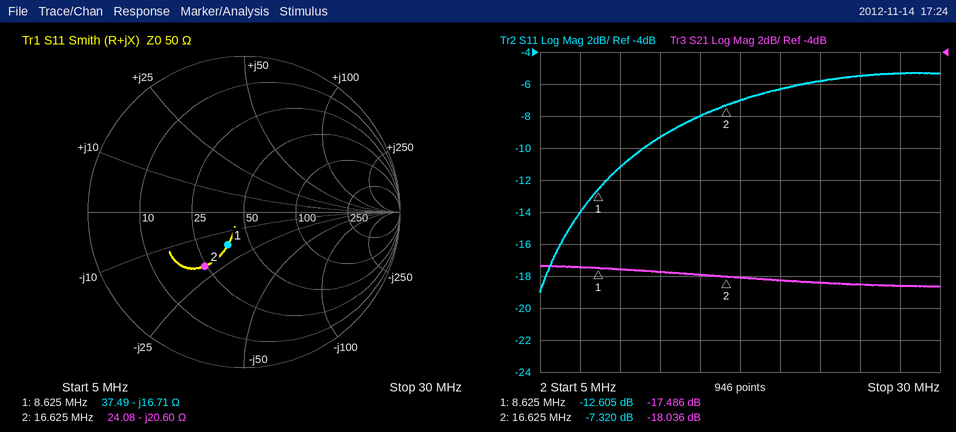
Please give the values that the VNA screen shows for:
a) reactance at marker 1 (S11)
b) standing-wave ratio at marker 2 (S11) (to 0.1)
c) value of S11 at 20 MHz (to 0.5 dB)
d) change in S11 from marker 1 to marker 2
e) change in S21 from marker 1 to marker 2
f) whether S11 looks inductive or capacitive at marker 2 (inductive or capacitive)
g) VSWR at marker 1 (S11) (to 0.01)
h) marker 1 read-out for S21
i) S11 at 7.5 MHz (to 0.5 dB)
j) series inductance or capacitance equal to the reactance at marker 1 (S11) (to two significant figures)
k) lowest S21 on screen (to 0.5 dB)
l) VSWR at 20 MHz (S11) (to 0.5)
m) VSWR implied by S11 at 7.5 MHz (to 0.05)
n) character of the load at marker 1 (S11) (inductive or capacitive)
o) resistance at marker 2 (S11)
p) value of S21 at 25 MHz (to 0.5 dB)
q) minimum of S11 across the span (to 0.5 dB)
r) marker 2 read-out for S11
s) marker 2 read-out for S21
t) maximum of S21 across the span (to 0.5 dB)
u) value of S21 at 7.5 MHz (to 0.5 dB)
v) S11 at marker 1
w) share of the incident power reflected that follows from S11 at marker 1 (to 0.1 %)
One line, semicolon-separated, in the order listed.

-16.71 Ω; 2.5; -6.5 dB; 5.285 dB; -0.550 dB; capacitive; 1.61; -17.486 dB; -14.0 dB; 1.1 nF; -18.5 dB; 3.0; 1.50; capacitive; 24.08 Ω; -18.5 dB; -19.0 dB; -7.320 dB; -18.036 dB; -17.5 dB; -17.5 dB; -12.605 dB; 5.5 %
